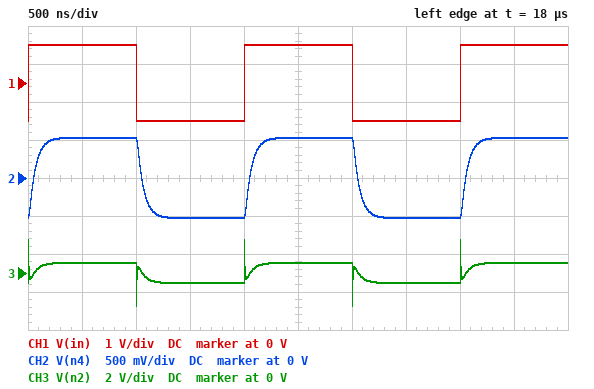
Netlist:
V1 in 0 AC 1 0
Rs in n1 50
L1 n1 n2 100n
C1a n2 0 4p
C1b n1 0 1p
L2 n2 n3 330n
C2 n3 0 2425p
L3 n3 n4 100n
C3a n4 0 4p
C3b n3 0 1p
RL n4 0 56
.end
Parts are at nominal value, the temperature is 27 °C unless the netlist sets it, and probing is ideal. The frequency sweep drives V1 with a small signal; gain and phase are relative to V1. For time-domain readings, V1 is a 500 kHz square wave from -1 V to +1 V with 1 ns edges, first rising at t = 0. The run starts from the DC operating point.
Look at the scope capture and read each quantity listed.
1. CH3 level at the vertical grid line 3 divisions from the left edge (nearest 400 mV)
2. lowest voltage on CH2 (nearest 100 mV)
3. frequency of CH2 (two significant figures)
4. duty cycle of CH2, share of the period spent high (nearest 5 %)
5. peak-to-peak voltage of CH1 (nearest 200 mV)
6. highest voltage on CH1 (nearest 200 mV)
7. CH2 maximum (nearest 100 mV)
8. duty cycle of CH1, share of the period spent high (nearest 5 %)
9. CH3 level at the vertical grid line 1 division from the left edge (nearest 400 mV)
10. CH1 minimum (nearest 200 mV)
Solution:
-400 mV
-500 mV
500 kHz
50 %
2.0 V
1.0 V
500 mV
50 %
400 mV
-1.0 V
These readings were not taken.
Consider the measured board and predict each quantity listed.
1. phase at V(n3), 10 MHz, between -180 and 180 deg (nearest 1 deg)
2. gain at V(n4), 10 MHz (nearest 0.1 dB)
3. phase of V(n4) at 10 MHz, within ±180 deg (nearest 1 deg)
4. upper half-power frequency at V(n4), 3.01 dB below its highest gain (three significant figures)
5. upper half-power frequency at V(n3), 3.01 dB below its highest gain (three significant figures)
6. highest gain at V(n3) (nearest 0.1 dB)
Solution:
-105 deg
-18.4 dB
-112 deg
2.67 MHz
2.67 MHz
-5.5 dB
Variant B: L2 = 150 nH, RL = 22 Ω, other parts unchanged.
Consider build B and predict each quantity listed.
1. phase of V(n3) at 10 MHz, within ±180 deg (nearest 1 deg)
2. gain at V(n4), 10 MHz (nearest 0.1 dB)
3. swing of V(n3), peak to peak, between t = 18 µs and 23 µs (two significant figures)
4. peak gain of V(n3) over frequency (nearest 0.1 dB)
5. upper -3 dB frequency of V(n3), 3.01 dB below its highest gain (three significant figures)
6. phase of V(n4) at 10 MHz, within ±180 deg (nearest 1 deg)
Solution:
-83 deg
-18.1 dB
610 mV
-10.3 dB
4.87 MHz
-99 deg
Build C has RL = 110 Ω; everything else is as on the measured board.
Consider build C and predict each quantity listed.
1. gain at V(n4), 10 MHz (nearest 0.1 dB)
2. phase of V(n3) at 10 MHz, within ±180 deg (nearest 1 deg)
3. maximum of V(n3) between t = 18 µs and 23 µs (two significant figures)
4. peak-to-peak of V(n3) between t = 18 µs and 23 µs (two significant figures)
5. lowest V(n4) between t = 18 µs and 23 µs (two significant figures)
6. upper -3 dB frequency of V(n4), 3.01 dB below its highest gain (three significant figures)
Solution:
-18.3 dB
-109 deg
690 mV
1.4 V
-690 mV
2.04 MHz
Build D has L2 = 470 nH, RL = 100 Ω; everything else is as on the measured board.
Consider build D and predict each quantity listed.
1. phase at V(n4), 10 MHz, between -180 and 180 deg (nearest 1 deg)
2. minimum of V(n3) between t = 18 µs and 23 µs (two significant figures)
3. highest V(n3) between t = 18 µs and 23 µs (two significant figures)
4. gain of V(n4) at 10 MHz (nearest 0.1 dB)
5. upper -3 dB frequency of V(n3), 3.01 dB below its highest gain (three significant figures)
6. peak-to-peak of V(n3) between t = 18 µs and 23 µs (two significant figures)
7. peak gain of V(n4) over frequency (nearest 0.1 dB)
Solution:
-120 deg
-670 mV
670 mV
-18.9 dB
2.15 MHz
1.3 V
-3.5 dB
